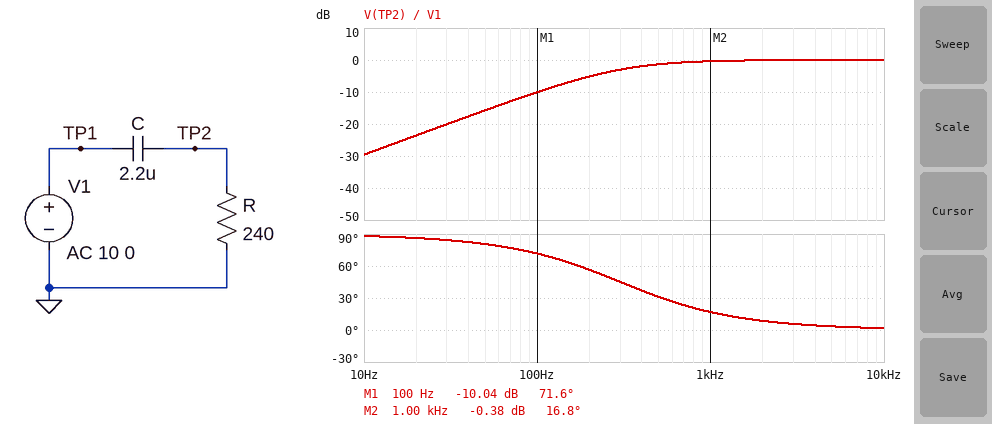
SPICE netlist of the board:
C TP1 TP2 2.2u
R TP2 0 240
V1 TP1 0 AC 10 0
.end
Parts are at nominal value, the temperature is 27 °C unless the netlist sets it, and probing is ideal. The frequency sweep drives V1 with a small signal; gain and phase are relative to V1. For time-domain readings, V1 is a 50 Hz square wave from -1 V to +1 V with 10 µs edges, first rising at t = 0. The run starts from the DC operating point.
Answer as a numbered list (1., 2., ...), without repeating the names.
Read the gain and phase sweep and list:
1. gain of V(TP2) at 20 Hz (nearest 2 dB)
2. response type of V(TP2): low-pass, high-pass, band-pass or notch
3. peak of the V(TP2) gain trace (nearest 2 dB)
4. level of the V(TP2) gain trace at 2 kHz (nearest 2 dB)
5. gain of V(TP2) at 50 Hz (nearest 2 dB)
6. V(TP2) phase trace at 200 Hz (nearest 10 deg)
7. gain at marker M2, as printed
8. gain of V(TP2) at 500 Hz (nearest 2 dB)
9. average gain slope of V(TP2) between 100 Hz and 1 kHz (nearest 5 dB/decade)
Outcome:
1. -24 dB
2. high-pass
3. 0 dB
4. 0 dB
5. -16 dB
6. 60 deg
7. -0.38 dB
8. -2 dB
9. 10 dB/decade
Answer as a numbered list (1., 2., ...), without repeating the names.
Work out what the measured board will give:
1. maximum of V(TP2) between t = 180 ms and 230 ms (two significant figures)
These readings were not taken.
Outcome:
1. 2.0 V
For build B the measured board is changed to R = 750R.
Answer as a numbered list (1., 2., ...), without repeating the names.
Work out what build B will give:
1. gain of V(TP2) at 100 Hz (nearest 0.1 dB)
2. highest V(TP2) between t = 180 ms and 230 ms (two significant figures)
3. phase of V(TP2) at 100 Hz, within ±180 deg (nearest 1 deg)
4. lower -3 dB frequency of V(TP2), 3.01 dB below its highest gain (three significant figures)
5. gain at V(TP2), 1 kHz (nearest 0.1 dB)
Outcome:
1. -2.9 dB
2. 2.0 V
3. 44 deg
4. 96.5 Hz
5. 0 dB
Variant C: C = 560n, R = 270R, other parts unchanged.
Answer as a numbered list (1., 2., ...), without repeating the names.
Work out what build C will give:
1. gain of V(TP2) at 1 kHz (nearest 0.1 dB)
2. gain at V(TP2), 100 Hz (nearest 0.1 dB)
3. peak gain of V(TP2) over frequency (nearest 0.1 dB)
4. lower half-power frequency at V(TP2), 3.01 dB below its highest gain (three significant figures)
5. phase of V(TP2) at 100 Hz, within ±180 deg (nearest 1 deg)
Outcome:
1. -3.2 dB
2. -20.5 dB
3. 0 dB
4. 1.05 kHz
5. 85 deg
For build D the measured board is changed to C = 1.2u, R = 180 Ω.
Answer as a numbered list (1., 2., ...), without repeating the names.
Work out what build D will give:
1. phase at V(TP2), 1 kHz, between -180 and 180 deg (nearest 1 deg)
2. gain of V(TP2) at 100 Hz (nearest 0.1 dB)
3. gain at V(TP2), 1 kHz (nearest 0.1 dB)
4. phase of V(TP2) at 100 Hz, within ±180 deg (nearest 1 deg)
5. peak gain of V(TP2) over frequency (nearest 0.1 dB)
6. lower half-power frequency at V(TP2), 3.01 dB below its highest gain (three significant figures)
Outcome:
1. 36 deg
2. -17.4 dB
3. -1.9 dB
4. 82 deg
5. 0 dB
6. 737 Hz
